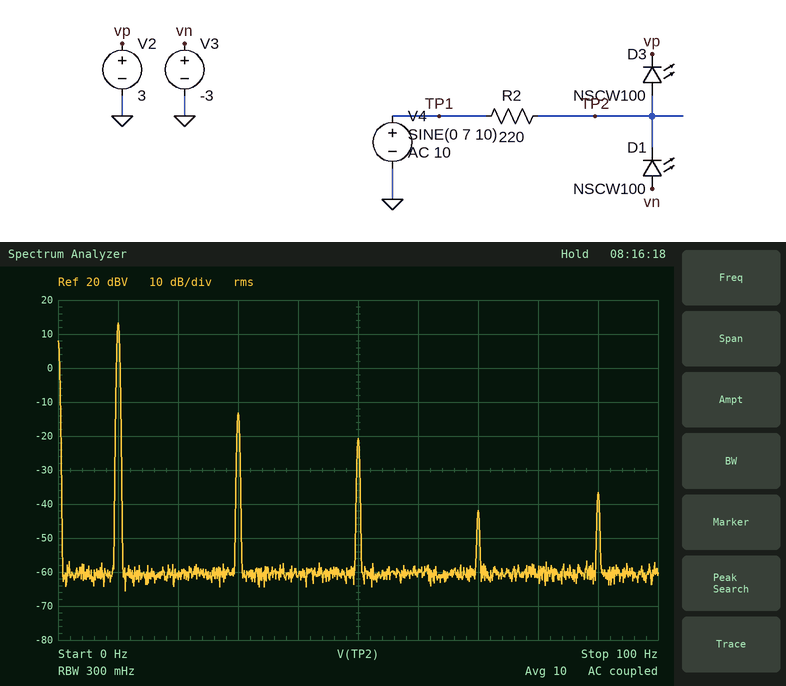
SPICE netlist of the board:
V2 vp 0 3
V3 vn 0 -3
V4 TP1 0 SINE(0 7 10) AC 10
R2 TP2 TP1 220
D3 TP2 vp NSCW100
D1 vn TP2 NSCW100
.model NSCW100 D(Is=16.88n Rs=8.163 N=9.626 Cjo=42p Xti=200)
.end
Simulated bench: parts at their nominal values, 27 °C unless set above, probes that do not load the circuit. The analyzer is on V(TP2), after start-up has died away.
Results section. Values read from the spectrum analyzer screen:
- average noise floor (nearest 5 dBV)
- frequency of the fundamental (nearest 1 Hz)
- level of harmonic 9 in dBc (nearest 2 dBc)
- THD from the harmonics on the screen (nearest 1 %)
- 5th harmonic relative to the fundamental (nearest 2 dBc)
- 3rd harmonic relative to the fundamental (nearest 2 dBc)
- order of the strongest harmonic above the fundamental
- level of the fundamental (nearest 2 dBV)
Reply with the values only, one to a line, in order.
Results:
-60 dBV
10 Hz
-50 dBc
5 %
-34 dBc
-26 dBc
3
14 dBV
